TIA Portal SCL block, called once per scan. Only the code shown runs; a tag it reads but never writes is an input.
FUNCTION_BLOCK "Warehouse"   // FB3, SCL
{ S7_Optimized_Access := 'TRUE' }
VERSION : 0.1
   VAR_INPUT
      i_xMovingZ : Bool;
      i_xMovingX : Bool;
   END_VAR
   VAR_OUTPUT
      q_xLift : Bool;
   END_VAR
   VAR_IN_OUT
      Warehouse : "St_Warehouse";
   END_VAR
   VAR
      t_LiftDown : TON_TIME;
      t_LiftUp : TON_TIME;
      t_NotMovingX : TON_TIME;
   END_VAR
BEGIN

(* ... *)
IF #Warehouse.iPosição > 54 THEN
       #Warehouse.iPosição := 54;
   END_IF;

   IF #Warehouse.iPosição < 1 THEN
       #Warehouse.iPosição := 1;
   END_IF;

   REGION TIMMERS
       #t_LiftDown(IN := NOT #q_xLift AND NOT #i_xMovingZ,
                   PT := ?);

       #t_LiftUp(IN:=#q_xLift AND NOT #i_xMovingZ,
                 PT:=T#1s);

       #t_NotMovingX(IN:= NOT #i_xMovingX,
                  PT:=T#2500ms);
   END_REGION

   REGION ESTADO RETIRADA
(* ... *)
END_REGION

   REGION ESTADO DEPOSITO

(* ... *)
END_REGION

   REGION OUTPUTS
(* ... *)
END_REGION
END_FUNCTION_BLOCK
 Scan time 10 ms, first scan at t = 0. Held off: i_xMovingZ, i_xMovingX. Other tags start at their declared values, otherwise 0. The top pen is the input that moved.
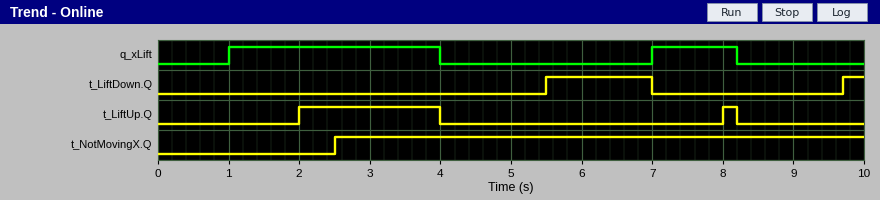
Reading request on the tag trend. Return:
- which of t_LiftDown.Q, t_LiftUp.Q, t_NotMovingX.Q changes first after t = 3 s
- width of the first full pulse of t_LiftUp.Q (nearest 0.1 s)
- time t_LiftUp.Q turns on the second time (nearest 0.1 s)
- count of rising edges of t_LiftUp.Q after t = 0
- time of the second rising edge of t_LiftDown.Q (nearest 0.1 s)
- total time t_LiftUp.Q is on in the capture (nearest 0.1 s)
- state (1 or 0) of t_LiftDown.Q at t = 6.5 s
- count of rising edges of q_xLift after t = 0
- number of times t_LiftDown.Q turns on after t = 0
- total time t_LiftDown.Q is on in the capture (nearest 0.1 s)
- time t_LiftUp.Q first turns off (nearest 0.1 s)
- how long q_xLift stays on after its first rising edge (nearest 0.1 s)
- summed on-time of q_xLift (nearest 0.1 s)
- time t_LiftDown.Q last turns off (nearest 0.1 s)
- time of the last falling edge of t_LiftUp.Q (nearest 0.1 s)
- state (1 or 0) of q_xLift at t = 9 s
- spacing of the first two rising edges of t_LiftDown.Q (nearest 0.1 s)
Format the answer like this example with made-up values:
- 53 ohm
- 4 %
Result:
- t_LiftUp.Q
- 2.0 s
- 8.0 s
- 2
- 9.7 s
- 2.2 s
- 1
- 2
- 2
- 1.8 s
- 4.0 s
- 3.0 s
- 4.2 s
- 7.0 s
- 8.2 s
- 0
- 4.2 s
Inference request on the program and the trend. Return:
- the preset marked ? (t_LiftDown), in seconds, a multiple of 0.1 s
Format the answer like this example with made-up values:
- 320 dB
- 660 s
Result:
- 1.5 s
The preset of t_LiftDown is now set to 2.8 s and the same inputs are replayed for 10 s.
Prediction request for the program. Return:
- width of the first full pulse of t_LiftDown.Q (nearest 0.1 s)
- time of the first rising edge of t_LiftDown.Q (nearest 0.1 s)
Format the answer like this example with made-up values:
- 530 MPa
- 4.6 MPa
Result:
- 0.2 s
- 6.8 s
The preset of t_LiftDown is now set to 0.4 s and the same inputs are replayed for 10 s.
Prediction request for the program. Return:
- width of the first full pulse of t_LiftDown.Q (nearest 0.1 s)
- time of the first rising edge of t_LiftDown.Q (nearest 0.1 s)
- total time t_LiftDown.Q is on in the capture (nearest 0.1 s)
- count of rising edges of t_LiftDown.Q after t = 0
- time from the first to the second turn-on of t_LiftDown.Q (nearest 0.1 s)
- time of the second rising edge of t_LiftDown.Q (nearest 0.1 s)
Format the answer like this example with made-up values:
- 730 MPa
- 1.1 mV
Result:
- 0.6 s
- 0.4 s
- 4.6 s
- 3
- 4.0 s
- 4.4 s
